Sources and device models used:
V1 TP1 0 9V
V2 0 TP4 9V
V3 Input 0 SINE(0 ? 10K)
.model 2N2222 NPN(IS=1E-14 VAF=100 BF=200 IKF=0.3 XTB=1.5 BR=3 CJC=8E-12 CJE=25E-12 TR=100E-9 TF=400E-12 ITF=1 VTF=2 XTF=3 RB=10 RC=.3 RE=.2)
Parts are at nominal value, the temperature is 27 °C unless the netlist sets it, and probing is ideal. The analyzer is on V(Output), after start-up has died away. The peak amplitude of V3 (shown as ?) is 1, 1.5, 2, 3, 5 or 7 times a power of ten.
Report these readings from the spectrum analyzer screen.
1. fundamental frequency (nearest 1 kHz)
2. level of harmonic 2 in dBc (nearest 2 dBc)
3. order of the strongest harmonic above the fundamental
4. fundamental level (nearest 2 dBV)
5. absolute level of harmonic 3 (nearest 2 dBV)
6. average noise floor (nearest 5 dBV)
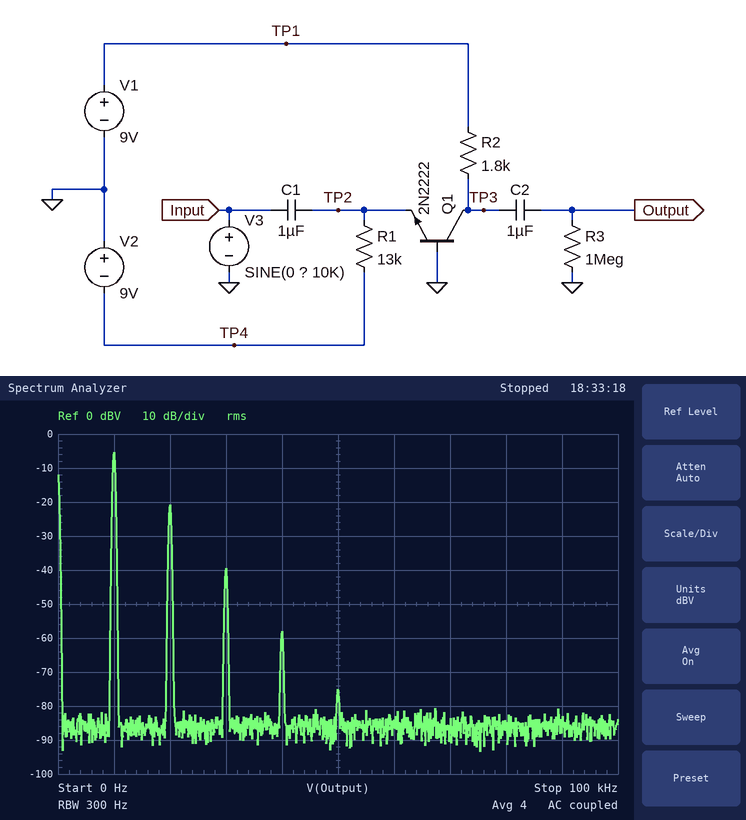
10 kHz
-16 dBc
2
-6 dBV
-40 dBV
-85 dBV
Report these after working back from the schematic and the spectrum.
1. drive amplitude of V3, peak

20 mV
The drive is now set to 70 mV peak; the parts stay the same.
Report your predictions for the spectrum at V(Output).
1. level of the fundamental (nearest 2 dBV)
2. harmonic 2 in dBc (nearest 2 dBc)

2 dBV
-6 dBc
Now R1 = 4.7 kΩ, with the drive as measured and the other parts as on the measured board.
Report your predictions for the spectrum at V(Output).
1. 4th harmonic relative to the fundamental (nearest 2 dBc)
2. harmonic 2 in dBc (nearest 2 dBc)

-56 dBc
-20 dBc
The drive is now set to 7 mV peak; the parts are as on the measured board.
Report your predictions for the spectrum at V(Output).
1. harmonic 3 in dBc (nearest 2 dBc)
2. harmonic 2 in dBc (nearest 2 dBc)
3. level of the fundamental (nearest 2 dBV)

-52 dBc
-24 dBc
-14 dBV
